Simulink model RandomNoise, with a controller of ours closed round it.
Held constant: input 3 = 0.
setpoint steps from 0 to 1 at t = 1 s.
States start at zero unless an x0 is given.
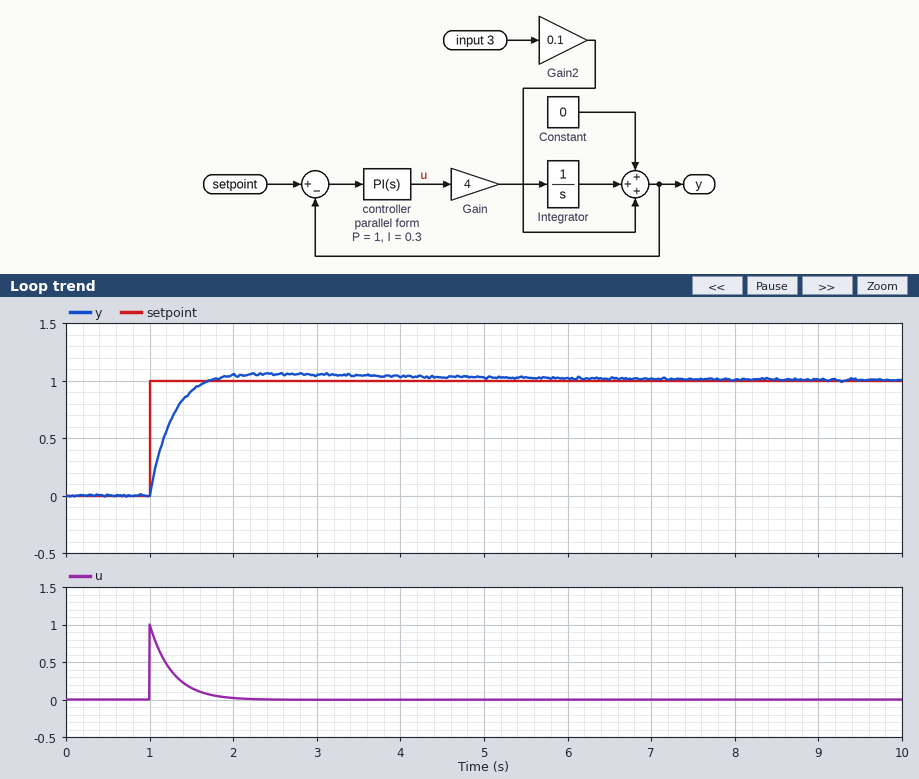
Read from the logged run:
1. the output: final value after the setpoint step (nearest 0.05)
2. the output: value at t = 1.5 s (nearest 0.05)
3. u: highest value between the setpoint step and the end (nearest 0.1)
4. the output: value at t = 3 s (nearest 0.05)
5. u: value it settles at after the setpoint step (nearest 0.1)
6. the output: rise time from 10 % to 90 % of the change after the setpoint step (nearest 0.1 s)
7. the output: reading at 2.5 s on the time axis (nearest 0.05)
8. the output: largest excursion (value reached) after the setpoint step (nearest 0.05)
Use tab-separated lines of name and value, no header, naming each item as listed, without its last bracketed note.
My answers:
the output: final value after the setpoint step	1.00
the output: value at t = 1.5 s	0.90
u: highest value between the setpoint step and the end	1.0
the output: value at t = 3 s	1.05
u: value it settles at after the setpoint step	0.0
the output: rise time from 10 % to 90 % of the change after the setpoint step	0.5 s
the output: reading at 2.5 s on the time axis	1.05
the output: largest excursion (value reached) after the setpoint step	1.05
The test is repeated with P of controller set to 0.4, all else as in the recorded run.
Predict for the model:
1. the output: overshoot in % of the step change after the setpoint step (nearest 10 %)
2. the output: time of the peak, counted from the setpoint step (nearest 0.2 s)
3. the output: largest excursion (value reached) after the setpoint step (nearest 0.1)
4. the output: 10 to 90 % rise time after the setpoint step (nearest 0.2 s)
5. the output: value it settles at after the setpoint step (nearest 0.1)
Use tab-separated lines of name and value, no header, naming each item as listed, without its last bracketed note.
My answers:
the output: overshoot in % of the step change after the setpoint step	20 %
the output: time of the peak, counted from the setpoint step	2.0 s
the output: largest excursion (value reached) after the setpoint step	1.2
the output: 10 to 90 % rise time after the setpoint step	0.8 s
the output: value it settles at after the setpoint step	1.0
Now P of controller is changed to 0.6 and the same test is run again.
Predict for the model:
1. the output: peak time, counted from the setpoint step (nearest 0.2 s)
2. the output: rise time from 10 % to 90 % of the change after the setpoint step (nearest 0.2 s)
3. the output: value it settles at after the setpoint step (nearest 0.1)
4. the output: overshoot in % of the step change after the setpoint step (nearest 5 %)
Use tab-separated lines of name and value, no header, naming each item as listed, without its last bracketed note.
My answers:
the output: peak time, counted from the setpoint step	1.8 s
the output: rise time from 10 % to 90 % of the change after the setpoint step	0.6 s
the output: value it settles at after the setpoint step	1.0
the output: overshoot in % of the step change after the setpoint step	10 %
